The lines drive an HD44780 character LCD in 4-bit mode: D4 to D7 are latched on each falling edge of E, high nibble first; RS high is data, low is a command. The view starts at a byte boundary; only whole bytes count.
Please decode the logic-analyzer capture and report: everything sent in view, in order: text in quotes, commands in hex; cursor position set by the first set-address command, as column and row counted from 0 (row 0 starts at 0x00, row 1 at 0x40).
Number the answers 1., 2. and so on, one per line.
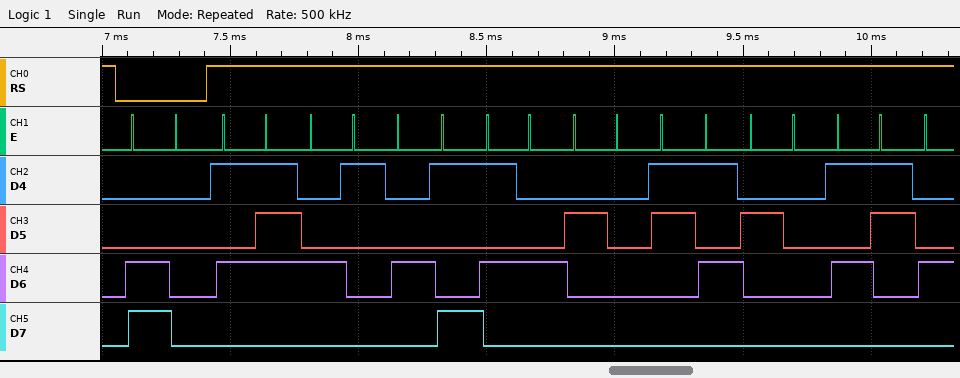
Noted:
1. 0xC0 "WAIT 5 S"
2. column 0, row 1
